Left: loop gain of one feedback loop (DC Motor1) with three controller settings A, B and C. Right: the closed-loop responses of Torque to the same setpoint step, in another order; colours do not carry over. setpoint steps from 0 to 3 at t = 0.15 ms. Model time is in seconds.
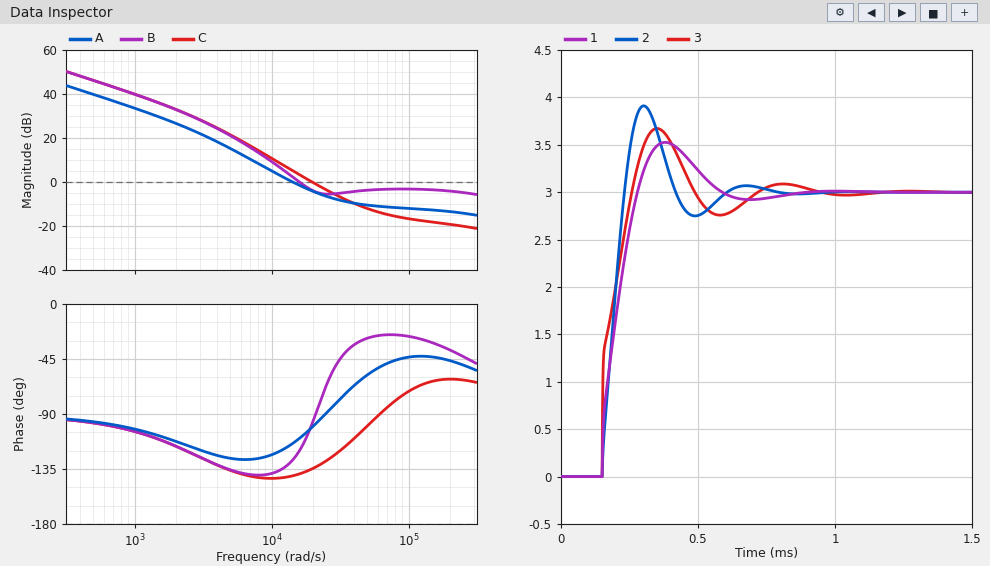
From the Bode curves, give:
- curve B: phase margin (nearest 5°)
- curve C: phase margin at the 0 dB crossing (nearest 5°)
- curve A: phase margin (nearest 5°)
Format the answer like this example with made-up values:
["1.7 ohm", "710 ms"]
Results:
["60°", "45°", "65°"]
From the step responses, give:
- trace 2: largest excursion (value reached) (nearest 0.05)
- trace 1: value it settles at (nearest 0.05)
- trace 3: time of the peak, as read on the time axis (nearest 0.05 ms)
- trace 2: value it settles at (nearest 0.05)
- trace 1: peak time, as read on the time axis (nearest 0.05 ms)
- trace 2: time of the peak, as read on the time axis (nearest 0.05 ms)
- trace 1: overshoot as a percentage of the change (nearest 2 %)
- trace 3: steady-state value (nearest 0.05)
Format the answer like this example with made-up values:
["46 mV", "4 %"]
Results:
["3.90", "3.00", "0.35 ms", "3.00", "0.40 ms", "0.30 ms", "18 %", "3.00"]
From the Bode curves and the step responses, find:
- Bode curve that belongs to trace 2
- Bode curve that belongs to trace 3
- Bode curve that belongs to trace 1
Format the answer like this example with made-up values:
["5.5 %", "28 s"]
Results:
["C", "B", "A"]
